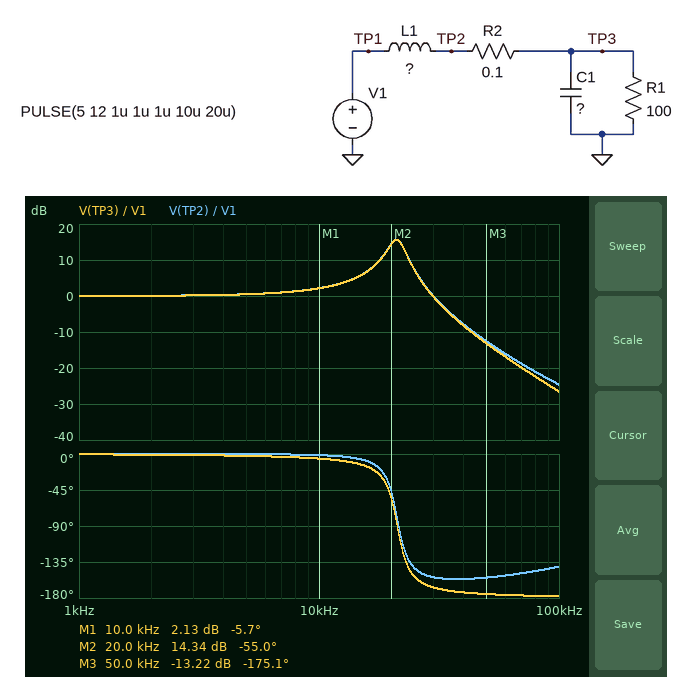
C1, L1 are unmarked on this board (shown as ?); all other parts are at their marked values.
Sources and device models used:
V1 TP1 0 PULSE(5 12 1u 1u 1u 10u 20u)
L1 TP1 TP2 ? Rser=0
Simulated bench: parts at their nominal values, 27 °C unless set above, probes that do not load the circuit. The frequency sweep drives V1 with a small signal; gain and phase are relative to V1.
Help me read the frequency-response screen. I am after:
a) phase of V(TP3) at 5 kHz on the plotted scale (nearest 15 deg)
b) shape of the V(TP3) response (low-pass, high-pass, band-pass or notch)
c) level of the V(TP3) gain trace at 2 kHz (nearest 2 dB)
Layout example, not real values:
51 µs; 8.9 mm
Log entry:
0 deg; low-pass; 0 dB
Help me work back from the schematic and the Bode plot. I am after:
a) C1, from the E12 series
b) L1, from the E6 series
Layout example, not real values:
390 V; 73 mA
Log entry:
12 µF; 4.7 µH
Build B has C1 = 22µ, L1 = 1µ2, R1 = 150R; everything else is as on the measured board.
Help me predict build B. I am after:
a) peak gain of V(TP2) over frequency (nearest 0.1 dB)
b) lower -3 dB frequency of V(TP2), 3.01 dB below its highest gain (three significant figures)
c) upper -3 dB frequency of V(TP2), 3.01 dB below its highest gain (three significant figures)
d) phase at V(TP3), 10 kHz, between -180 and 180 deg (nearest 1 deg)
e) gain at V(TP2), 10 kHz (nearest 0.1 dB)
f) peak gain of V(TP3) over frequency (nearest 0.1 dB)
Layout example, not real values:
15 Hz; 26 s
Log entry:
8.2 dB; 22.2 kHz; 36.1 kHz; -9 deg; 0.9 dB; 7.5 dB
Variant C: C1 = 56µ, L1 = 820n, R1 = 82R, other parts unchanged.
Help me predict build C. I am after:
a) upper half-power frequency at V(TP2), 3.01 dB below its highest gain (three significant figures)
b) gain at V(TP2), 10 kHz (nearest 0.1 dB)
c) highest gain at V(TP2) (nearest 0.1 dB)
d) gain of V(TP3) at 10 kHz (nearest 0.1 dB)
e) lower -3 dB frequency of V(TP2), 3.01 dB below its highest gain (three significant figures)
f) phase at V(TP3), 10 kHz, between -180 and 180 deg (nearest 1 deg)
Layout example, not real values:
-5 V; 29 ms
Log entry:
30.6 kHz; 1.5 dB; 4.2 dB; 1.0 dB; 8.85 kHz; -23 deg
